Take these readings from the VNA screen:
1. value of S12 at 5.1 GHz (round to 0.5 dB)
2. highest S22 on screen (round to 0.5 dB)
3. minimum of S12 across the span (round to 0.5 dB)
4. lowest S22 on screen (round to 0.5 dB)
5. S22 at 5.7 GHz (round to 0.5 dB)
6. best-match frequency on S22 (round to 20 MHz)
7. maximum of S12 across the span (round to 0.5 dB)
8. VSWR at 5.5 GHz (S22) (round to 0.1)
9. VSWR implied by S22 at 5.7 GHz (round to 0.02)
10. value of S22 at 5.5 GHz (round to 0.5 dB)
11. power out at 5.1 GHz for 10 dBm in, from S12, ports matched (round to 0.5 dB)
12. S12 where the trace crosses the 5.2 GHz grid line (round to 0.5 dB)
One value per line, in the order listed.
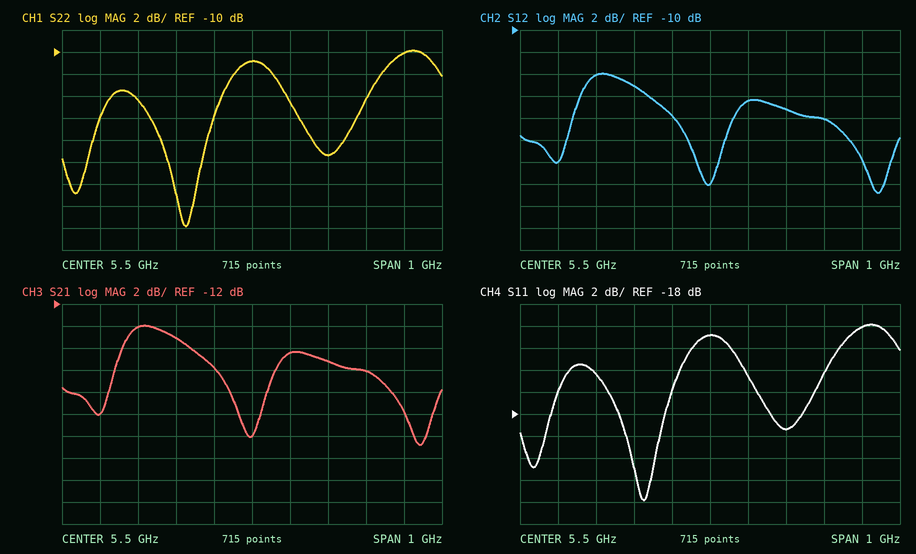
-22.0 dB
-10.0 dB
-25.0 dB
-26.0 dB
-19.5 dB
5.32 GHz
-14.0 dB
1.8
1.24
-11.0 dB
-12.0 dBm
-14.0 dB
